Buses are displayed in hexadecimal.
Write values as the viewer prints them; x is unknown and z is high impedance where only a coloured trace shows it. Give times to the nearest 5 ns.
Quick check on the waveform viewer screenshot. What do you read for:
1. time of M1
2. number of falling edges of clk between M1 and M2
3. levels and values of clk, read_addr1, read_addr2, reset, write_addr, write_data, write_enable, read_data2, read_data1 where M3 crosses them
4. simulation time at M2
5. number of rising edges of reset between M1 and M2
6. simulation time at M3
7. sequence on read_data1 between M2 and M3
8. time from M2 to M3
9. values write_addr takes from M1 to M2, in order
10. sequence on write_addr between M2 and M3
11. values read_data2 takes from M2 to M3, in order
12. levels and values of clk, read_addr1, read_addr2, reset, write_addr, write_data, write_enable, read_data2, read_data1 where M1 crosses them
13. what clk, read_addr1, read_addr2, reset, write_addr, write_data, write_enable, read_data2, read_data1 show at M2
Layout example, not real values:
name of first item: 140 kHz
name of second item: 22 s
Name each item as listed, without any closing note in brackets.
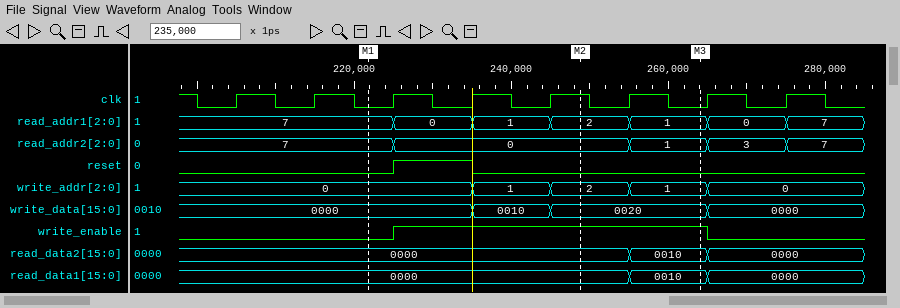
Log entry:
time of M1: 220 ns
number of falling edges of clk between M1 and M2: 2
levels and values of clk, read_addr1, read_addr2, reset, write_addr, write_data, write_enable, read_data2, read_data1 where M3 crosses them: clk=0, read_addr1=1, read_addr2=1, reset=0, write_addr=1, write_data=0020, write_enable=1, read_data2=0010, read_data1=0010
simulation time at M2: 250 ns
number of rising edges of reset between M1 and M2: 1
simulation time at M3: 265 ns
sequence on read_data1 between M2 and M3: 0000, 0010
time from M2 to M3: 15 ns
values write_addr takes from M1 to M2, in order: 0, 1, 2
sequence on write_addr between M2 and M3: 2, 1
values read_data2 takes from M2 to M3, in order: 0000, 0010
levels and values of clk, read_addr1, read_addr2, reset, write_addr, write_data, write_enable, read_data2, read_data1 where M1 crosses them: clk=0, read_addr1=7, read_addr2=7, reset=0, write_addr=0, write_data=0000, write_enable=0, read_data2=0000, read_data1=0000
what clk, read_addr1, read_addr2, reset, write_addr, write_data, write_enable, read_data2, read_data1 show at M2: clk=1, read_addr1=2, read_addr2=0, reset=0, write_addr=2, write_data=0020, write_enable=1, read_data2=0000, read_data1=0000
